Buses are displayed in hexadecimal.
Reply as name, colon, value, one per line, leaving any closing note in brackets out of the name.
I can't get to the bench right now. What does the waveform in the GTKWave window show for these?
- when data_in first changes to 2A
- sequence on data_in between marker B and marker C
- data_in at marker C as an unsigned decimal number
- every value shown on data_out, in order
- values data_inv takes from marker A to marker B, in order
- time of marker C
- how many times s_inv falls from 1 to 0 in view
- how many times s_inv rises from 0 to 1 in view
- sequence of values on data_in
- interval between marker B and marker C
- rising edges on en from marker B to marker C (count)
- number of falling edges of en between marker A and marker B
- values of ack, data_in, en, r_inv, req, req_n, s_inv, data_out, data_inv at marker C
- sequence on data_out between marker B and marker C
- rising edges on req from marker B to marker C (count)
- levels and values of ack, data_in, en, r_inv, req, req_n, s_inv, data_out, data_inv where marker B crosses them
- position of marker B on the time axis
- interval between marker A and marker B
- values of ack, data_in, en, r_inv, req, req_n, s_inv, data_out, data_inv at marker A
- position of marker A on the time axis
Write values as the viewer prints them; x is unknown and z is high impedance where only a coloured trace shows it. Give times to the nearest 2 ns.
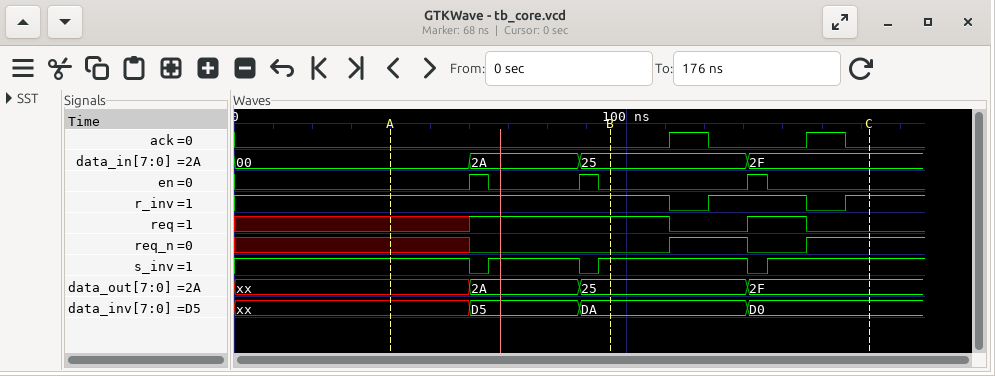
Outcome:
when data_in first changes to 2A: 60 ns
sequence on data_in between marker B and marker C: 25, 2F
data_in at marker C as an unsigned decimal number: 47
every value shown on data_out, in order: xx, 2A, 25, 2F
values data_inv takes from marker A to marker B, in order: xx, D5, DA
time of marker C: 162 ns
how many times s_inv falls from 1 to 0 in view: 3
how many times s_inv rises from 0 to 1 in view: 3
sequence of values on data_in: 00, 2A, 25, 2F
interval between marker B and marker C: 66 ns
rising edges on en from marker B to marker C: 1
number of falling edges of en between marker A and marker B: 2
values of ack, data_in, en, r_inv, req, req_n, s_inv, data_out, data_inv at marker C: ack=0, data_in=2F, en=0, r_inv=1, req=0, req_n=1, s_inv=1, data_out=2F, data_inv=D0
sequence on data_out between marker B and marker C: 25, 2F
rising edges on req from marker B to marker C: 1
levels and values of ack, data_in, en, r_inv, req, req_n, s_inv, data_out, data_inv where marker B crosses them: ack=0, data_in=25, en=0, r_inv=1, req=1, req_n=0, s_inv=1, data_out=25, data_inv=DA
position of marker B on the time axis: 96 ns
interval between marker A and marker B: 56 ns
values of ack, data_in, en, r_inv, req, req_n, s_inv, data_out, data_inv at marker A: ack=0, data_in=00, en=0, r_inv=1, req=x, req_n=x, s_inv=1, data_out=xx, data_inv=xx
position of marker A on the time axis: 40 ns
